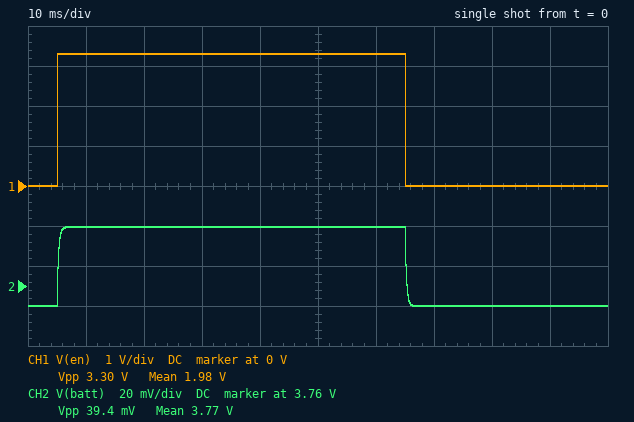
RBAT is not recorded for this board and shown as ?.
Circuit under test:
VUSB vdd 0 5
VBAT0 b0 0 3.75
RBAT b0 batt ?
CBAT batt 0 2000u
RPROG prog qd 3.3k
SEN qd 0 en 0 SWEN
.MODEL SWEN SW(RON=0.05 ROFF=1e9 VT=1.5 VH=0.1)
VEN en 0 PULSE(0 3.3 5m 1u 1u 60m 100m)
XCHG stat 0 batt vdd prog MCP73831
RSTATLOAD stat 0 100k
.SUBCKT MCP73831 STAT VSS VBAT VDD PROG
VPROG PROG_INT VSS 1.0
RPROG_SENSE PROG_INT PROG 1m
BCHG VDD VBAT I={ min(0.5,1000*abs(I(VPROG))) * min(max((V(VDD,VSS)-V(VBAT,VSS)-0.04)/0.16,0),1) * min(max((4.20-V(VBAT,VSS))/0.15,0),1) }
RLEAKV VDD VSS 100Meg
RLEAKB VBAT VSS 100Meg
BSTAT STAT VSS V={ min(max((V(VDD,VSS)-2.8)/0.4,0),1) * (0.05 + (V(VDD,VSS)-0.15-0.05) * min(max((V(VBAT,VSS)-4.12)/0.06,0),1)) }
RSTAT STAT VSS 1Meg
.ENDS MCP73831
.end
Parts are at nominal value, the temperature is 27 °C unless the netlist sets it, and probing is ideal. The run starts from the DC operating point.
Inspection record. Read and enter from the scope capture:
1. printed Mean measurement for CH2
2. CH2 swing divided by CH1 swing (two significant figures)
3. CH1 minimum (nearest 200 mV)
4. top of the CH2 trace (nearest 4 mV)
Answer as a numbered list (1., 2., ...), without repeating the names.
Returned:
1. 3.77 V
2. 0.012
3. 0 V
4. 3.788 V
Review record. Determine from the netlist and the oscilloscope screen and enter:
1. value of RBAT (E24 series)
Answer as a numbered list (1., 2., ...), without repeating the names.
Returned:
1. 0.13 Ω
